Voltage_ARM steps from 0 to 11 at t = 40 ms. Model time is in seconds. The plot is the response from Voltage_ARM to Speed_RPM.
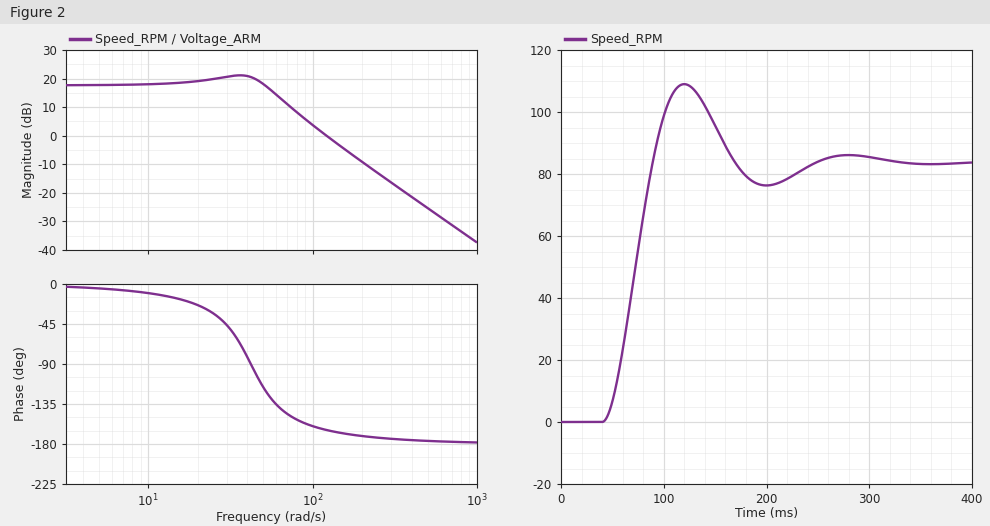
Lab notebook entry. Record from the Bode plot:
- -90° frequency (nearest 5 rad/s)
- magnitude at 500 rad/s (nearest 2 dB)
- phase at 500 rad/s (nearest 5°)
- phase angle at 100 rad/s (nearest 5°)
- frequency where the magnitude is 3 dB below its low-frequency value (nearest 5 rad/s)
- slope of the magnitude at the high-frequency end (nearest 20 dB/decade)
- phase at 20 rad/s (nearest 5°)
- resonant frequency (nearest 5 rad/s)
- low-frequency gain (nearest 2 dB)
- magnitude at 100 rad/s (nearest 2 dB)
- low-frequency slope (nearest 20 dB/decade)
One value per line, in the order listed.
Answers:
40 rad/s
-26 dB
-175°
-160°
60 rad/s
-40 dB/decade
-25°
35 rad/s
18 dB
4 dB
0 dB/decade
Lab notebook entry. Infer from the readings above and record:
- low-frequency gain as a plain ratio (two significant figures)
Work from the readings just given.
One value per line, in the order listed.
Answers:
7.9
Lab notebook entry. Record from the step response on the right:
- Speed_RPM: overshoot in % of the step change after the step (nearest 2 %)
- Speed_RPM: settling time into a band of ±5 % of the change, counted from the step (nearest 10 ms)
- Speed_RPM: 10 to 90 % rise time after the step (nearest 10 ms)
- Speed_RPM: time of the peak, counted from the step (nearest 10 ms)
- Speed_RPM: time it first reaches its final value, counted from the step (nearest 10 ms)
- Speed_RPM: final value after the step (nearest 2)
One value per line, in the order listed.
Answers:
30 %
190 ms
30 ms
80 ms
50 ms
84
